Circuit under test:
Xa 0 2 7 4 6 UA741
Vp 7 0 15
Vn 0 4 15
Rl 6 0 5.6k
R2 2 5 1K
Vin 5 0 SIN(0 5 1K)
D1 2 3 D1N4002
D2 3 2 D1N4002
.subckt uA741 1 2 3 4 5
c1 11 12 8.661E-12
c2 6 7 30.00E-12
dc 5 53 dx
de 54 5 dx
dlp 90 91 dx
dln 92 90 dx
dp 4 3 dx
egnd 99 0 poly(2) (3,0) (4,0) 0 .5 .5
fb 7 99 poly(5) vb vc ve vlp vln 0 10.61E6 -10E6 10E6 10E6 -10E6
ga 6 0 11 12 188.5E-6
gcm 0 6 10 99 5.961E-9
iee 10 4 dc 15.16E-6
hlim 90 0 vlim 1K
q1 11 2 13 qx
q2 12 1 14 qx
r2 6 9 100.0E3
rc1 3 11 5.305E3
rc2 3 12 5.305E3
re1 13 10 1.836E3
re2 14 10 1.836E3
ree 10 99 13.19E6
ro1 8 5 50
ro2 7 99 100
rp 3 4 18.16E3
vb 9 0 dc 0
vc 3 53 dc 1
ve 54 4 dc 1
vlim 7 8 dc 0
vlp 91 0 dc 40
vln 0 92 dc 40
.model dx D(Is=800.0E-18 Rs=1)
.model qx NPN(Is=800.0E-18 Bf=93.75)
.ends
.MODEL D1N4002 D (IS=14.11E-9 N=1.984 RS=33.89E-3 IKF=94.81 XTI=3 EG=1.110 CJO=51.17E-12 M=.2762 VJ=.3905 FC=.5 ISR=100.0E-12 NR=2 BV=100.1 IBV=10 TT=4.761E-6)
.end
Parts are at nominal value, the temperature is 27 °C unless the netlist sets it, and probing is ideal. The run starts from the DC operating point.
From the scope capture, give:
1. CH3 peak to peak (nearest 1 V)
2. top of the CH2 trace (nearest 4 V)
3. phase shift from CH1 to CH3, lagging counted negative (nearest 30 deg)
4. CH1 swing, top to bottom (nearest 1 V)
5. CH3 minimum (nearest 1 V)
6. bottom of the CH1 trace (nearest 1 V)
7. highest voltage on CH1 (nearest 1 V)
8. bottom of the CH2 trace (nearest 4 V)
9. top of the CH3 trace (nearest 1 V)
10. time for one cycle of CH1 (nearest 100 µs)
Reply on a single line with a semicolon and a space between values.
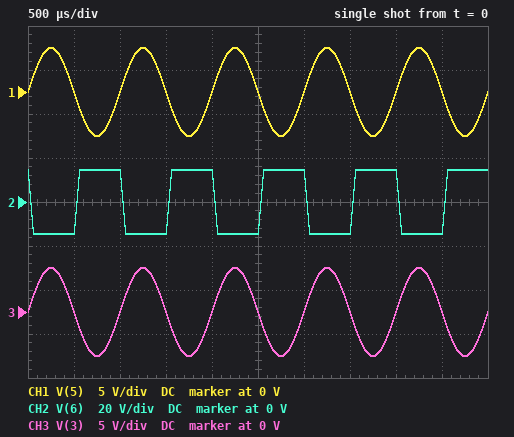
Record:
10 V; 16 V; 0 deg; 10 V; -5 V; -5 V; 5 V; -16 V; 5 V; 1.0 ms
